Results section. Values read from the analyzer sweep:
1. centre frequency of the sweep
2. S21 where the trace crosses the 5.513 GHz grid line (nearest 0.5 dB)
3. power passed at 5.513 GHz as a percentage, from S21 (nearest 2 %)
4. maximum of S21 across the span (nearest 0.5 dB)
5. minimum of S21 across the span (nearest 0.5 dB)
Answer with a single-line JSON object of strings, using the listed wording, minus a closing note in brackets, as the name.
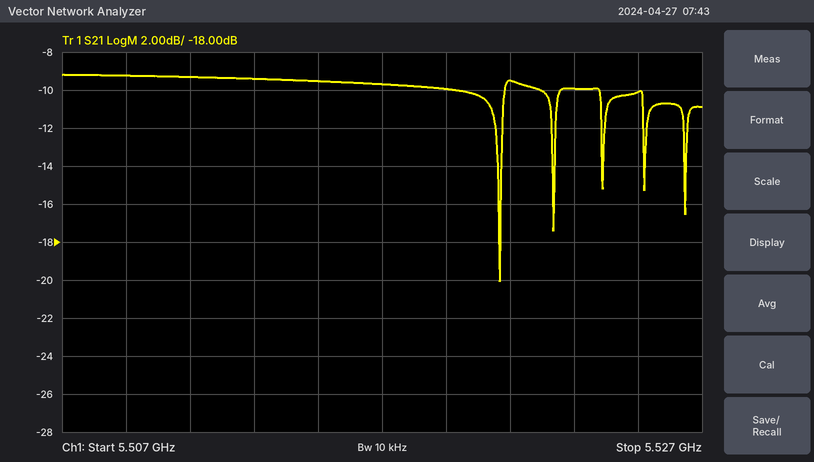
{"centre frequency of the sweep": "5.517 GHz", "S21 where the trace crosses the 5.513 GHz grid line": "-9.5 dB", "power passed at 5.513 GHz as a percentage, from S21": "12 %", "maximum of S21 across the span": "-9.0 dB", "minimum of S21 across the span": "-20.0 dB"}
